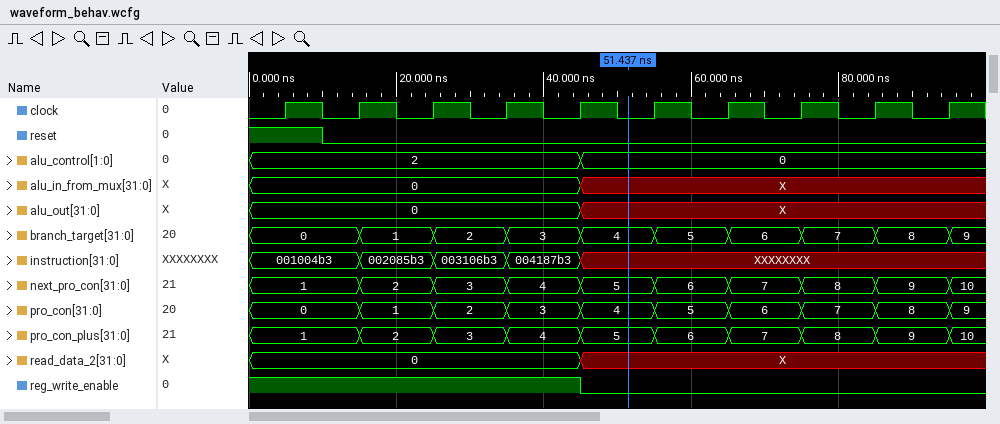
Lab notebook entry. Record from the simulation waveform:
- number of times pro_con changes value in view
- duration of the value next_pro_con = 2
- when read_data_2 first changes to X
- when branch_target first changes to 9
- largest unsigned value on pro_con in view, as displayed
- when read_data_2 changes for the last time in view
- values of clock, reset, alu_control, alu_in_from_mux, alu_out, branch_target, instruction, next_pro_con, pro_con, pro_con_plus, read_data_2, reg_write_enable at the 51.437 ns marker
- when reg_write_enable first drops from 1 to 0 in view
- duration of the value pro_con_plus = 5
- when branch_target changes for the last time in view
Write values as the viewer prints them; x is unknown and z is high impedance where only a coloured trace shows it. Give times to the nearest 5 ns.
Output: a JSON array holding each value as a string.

["9", "10 ns", "45 ns", "95 ns", "9", "45 ns", "clock=0, reset=0, alu_control=0, alu_in_from_mux=X, alu_out=X, branch_target=4, instruction=XXXXXXXX, next_pro_con=5, pro_con=4, pro_con_plus=5, read_data_2=X, reg_write_enable=0", "45 ns", "10 ns", "95 ns"]
